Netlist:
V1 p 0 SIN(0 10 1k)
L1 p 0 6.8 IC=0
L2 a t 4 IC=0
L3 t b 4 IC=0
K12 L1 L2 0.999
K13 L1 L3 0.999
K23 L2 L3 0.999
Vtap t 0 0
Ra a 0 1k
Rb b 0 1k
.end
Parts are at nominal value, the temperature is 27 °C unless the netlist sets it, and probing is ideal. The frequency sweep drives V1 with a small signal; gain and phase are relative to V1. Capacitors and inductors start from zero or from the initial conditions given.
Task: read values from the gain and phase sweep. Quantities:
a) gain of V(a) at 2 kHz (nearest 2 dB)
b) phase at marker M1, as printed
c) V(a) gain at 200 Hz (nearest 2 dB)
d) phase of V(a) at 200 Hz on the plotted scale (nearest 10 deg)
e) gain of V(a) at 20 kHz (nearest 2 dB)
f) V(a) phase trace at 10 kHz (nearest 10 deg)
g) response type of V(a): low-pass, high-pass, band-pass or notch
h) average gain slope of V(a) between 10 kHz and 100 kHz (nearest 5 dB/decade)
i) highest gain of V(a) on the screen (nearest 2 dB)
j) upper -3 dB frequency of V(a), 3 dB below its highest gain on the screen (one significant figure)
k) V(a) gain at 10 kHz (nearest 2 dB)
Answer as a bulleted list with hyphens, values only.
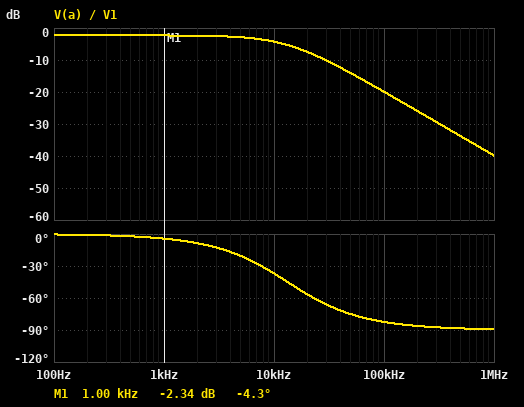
- -2 dB
- -4.3 deg
- -2 dB
- 0 deg
- -8 dB
- -40 deg
- low-pass
- -15 dB/decade
- -2 dB
- 10 kHz
- -4 dB
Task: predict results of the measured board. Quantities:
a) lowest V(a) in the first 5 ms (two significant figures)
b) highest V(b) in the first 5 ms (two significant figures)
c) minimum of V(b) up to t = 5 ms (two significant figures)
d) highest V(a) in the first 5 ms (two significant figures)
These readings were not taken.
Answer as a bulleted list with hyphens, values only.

- -7.6 V
- 7.6 V
- -7.6 V
- 7.6 V
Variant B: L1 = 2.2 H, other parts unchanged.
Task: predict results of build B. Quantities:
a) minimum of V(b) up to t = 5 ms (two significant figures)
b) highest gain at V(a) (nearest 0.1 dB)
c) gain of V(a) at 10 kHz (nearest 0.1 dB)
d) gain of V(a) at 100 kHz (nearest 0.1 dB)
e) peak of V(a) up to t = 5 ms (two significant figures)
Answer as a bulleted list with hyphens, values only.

- -13 V
- 2.6 dB
- 0.6 dB
- -15.0 dB
- 13 V
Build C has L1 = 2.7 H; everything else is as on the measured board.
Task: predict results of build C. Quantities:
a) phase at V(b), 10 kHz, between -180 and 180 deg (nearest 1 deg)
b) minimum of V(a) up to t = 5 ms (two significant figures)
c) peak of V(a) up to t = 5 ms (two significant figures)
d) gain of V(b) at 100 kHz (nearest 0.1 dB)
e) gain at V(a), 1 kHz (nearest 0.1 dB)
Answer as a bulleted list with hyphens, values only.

- 143 deg
- -12 V
- 12 V
- -15.9 dB
- 1.7 dB
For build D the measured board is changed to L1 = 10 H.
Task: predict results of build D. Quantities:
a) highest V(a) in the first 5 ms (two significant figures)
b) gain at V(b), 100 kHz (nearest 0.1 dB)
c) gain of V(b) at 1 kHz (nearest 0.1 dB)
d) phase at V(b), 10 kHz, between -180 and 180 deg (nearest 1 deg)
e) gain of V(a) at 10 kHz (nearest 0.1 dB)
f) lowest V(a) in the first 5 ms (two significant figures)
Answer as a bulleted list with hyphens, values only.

- 6.3 V
- -21.6 dB
- -4.0 dB
- 143 deg
- -5.9 dB
- -6.3 V
